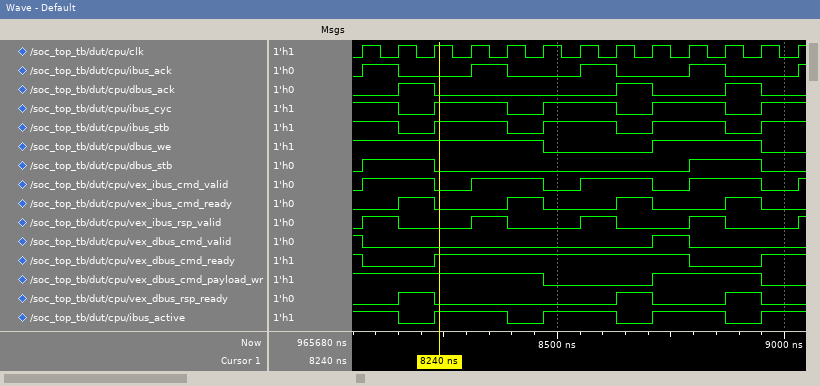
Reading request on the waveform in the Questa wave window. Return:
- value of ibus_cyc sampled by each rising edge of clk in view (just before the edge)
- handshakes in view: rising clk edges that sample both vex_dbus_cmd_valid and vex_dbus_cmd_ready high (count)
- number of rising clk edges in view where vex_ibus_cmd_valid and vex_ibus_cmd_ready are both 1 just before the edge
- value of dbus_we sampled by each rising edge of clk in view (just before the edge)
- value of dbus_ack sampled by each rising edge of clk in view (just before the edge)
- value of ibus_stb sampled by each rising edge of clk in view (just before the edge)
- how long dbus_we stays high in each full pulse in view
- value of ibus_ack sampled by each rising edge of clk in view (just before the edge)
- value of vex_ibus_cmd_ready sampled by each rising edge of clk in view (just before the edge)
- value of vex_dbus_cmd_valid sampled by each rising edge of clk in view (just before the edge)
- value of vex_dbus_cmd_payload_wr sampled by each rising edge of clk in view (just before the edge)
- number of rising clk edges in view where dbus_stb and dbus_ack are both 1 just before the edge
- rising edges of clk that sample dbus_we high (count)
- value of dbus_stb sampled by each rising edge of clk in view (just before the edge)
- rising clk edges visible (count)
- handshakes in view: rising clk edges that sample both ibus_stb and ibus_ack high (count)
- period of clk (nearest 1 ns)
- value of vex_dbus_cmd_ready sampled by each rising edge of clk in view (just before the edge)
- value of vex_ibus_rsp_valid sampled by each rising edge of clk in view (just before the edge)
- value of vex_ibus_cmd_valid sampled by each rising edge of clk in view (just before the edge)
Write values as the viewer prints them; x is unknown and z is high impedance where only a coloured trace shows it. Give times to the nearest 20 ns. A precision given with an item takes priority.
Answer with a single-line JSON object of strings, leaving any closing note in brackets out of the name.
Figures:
{"value of ibus_cyc sampled by each rising edge of clk in view": "1 1 0 1 1 0 1 1 0 1 1 0 1", "handshakes in view: rising clk edges that sample both vex_dbus_cmd_valid and vex_dbus_cmd_ready high": "2", "number of rising clk edges in view where vex_ibus_cmd_valid and vex_ibus_cmd_ready are both 1 just before the edge": "4", "value of dbus_we sampled by each rising edge of clk in view": "1 1 1 1 1 1 0 0 0 1 1 1 0", "value of dbus_ack sampled by each rising edge of clk in view": "0 0 1 0 0 0 0 0 1 0 0 1 0", "value of ibus_stb sampled by each rising edge of clk in view": "1 1 0 1 1 0 1 1 0 1 1 0 1", "how long dbus_we stays high in each full pulse in view": "240 ns", "value of ibus_ack sampled by each rising edge of clk in view": "0 1 0 0 1 0 0 1 0 0 1 0 0", "value of vex_ibus_cmd_ready sampled by each rising edge of clk in view": "0 0 1 0 0 1 0 0 1 0 0 1 0", "value of vex_dbus_cmd_valid sampled by each rising edge of clk in view": "1 0 0 0 0 0 0 0 0 1 0 0 0", "value of vex_dbus_cmd_payload_wr sampled by each rising edge of clk in view": "1 1 1 1 1 1 0 0 0 1 1 1 0", "number of rising clk edges in view where dbus_stb and dbus_ack are both 1 just before the edge": "2", "rising edges of clk that sample dbus_we high": "9", "value of dbus_stb sampled by each rising edge of clk in view": "0 1 1 0 0 0 0 0 0 0 1 1 0", "rising clk edges visible": "13", "handshakes in view: rising clk edges that sample both ibus_stb and ibus_ack high": "4", "period of clk": "80 ns", "value of vex_dbus_cmd_ready sampled by each rising edge of clk in view": "1 0 0 1 1 1 1 1 1 1 0 0 1", "value of vex_ibus_rsp_valid sampled by each rising edge of clk in view": "0 1 0 0 1 0 0 1 0 0 1 0 0", "value of vex_ibus_cmd_valid sampled by each rising edge of clk in view": "0 1 1 0 1 1 0 1 1 0 1 1 0"}
